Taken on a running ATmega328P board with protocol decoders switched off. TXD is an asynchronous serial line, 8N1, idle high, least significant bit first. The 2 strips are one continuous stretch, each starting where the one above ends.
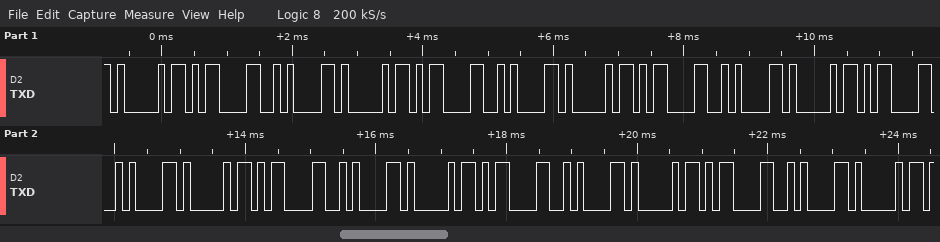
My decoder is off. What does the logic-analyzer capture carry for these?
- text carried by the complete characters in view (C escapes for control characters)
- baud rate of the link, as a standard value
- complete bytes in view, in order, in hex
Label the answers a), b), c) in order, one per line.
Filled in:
a) "A\r\nA\r\nA\r\nA\r\nA\r\nA\r\nA\r\nA"
b) 9600 baud
c) 41 0D 0A 41 0D 0A 41 0D 0A 41 0D 0A 41 0D 0A 41 0D 0A 41 0D 0A 41
